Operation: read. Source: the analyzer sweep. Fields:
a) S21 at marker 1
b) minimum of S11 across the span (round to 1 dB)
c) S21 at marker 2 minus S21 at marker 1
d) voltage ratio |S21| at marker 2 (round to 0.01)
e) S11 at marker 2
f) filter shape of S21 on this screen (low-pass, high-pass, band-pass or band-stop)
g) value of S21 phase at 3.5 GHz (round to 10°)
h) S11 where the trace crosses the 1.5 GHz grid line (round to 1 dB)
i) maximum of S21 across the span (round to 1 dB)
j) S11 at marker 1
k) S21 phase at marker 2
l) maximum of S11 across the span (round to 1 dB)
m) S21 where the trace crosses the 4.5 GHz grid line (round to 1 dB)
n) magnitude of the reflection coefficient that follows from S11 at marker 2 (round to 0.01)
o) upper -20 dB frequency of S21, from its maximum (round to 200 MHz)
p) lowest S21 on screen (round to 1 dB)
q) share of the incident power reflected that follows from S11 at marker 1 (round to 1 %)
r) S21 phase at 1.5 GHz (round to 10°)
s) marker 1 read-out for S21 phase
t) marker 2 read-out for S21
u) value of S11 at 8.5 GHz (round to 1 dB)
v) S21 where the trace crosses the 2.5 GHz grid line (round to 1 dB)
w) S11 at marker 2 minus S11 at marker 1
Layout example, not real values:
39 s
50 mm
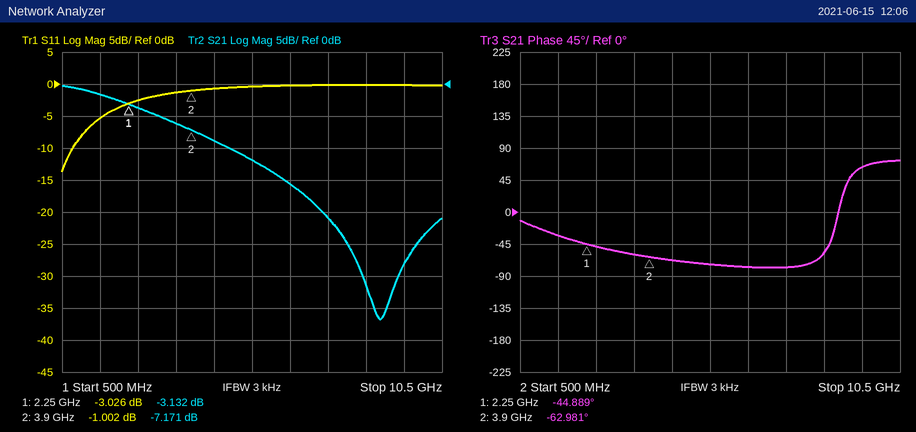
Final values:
-3.132 dB
-14 dB
-4.039 dB
0.44
-1.002 dB
low-pass
-60°
-5 dB
0 dB
-3.026 dB
-62.981°
0 dB
-9 dB
0.89
7.4 GHz
-37 dB
50 %
-30°
-44.889°
-7.171 dB
0 dB
-4 dB
2.024 dB
